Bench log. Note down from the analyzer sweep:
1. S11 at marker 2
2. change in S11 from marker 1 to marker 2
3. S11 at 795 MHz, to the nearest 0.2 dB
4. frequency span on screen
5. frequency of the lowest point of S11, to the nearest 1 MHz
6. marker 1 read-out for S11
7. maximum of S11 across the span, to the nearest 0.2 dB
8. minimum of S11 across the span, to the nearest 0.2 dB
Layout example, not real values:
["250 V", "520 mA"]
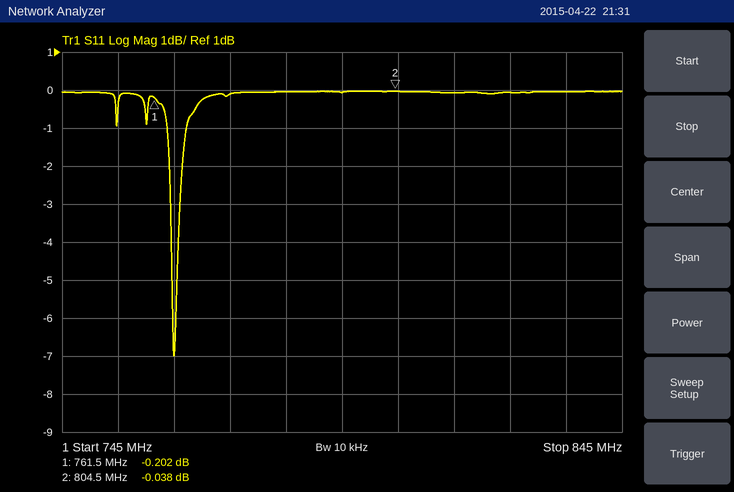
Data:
["-0.038 dB", "0.164 dB", "0.0 dB", "100 MHz", "765 MHz", "-0.202 dB", "0.0 dB", "-7.0 dB"]
